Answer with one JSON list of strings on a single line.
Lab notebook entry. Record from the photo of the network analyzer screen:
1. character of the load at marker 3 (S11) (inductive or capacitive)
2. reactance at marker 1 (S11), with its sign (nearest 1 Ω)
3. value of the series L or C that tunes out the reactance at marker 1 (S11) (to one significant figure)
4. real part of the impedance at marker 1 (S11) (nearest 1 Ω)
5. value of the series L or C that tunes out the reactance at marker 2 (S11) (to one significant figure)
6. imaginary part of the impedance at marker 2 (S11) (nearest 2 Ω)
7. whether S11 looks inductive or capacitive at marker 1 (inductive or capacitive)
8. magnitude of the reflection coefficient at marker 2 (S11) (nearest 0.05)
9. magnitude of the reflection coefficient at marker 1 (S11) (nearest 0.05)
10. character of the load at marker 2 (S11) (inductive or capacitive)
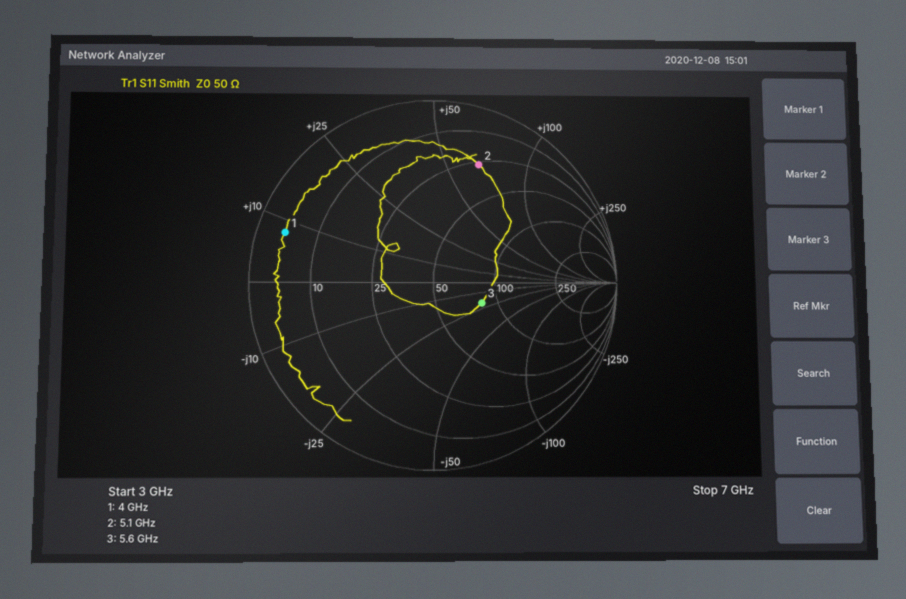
["capacitive", "+8 Ω", "5 pF", "4 Ω", "500 fF", "+66 Ω", "inductive", "0.70", "0.85", "inductive"]
